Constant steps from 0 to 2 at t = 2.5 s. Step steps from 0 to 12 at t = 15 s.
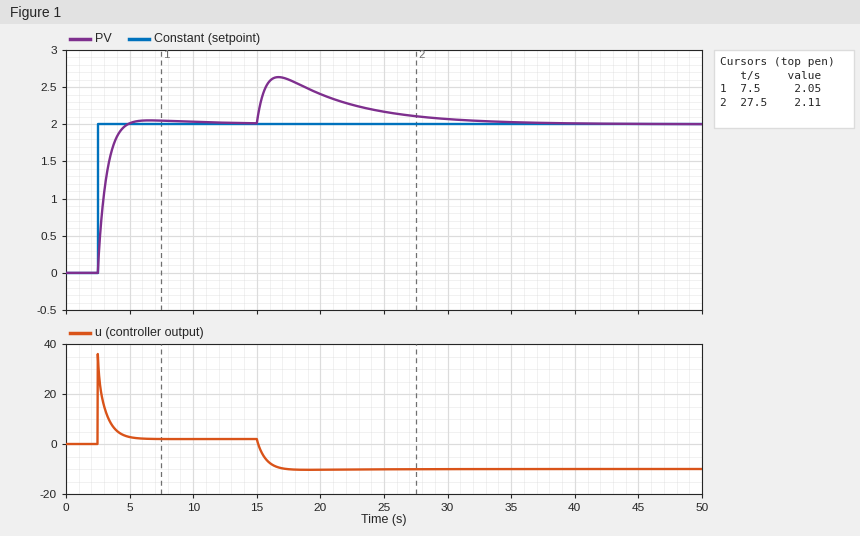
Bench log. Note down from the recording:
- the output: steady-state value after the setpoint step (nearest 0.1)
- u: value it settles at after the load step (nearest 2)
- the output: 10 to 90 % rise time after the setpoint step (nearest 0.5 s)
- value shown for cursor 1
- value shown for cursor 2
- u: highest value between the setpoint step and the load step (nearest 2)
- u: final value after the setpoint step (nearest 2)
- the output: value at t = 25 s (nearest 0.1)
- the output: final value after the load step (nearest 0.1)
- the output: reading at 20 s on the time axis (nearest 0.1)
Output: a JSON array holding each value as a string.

["2.0", "-10", "1.5 s", "2.05", "2.11", "36", "2", "2.2", "2.0", "2.4"]
